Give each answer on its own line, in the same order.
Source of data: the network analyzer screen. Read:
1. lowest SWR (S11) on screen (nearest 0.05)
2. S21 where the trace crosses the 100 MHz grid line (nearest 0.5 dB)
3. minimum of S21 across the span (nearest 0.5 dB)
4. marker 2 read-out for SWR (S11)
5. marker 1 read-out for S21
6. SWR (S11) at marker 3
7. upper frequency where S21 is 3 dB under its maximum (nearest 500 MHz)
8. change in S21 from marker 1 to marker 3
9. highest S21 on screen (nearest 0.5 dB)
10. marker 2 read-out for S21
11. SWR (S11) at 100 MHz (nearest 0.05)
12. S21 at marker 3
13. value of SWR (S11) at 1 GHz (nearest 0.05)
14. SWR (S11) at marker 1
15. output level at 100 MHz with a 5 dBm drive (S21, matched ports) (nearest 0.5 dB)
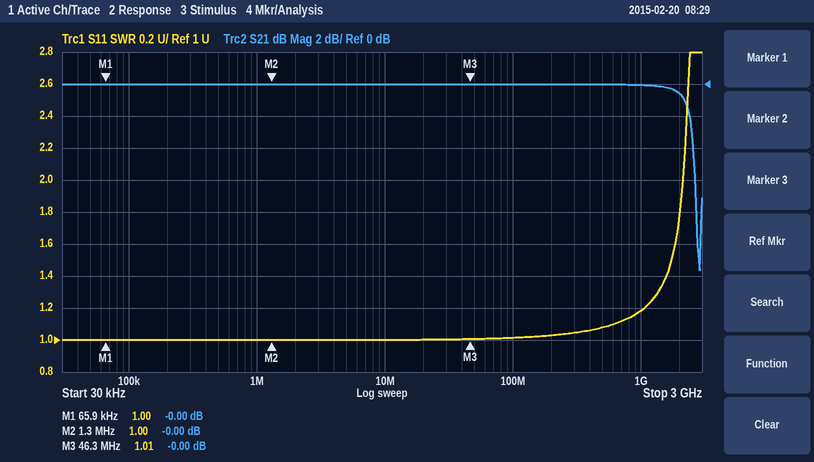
1.00
0.0 dB
-11.5 dB
1.00
-0.00 dB
1.01
2.5 GHz
0.00 dB
0.0 dB
-0.00 dB
1.00
-0.00 dB
1.20
1.00
5.0 dBm
